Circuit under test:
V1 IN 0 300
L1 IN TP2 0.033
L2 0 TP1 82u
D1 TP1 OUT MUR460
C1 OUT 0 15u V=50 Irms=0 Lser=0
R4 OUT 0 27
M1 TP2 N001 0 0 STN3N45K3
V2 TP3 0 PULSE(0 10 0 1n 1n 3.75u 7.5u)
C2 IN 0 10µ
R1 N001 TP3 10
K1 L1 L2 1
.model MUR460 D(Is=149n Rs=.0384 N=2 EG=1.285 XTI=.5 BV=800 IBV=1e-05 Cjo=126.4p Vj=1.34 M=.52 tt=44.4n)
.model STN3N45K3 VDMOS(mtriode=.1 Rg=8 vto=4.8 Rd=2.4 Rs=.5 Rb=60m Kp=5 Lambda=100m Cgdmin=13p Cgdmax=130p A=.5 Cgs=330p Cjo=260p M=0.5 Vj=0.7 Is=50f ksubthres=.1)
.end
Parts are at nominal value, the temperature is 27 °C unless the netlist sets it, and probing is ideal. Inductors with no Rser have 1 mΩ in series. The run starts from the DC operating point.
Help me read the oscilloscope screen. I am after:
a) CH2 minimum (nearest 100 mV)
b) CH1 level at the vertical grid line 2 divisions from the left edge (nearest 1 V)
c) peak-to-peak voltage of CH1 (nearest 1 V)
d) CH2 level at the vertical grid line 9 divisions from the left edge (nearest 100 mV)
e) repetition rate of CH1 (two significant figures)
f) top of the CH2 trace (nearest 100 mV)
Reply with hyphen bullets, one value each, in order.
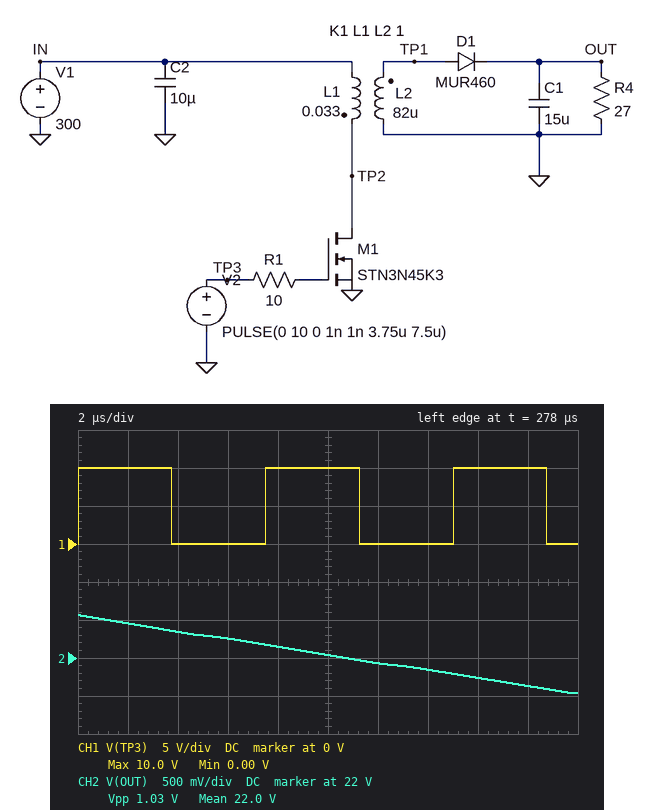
- 21.5 V
- 0 V
- 10 V
- 21.6 V
- 130 kHz
- 22.6 V
